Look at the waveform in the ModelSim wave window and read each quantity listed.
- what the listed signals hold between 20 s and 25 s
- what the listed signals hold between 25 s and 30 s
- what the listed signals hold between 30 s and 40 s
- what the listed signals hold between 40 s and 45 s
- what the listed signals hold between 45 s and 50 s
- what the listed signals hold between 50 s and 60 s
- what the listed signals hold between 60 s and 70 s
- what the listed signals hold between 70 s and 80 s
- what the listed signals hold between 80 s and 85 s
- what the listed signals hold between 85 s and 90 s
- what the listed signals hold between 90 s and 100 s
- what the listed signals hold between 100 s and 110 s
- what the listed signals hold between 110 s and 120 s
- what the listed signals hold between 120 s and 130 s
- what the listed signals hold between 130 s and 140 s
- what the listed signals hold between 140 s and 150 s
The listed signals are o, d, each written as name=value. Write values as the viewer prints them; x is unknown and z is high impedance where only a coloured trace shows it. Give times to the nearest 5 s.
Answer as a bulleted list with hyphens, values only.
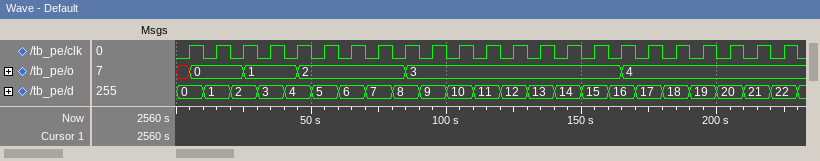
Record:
- o=0, d=2
- o=1, d=2
- o=1, d=3
- o=1, d=4
- o=2, d=4
- o=2, d=5
- o=2, d=6
- o=2, d=7
- o=2, d=8
- o=3, d=8
- o=3, d=9
- o=3, d=10
- o=3, d=11
- o=3, d=12
- o=3, d=13
- o=3, d=14
